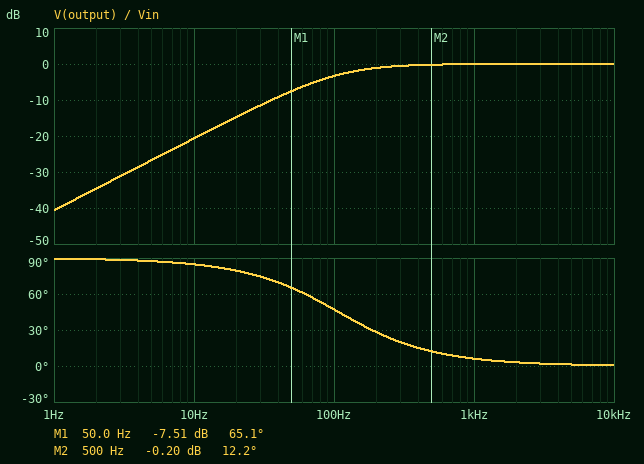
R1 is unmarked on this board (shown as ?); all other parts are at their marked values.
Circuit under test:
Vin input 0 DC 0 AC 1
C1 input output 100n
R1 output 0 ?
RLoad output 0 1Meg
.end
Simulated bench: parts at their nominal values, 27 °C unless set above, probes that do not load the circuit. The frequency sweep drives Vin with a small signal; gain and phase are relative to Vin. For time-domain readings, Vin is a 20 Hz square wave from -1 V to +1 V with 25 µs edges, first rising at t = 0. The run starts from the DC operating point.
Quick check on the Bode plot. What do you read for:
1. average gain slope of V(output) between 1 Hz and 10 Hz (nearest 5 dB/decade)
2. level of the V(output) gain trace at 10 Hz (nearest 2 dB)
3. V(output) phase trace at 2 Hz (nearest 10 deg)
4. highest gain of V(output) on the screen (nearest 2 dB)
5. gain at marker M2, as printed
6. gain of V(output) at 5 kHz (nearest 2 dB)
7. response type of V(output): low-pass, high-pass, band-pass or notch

20 dB/decade
-20 dB
90 deg
0 dB
-0.20 dB
0 dB
high-pass
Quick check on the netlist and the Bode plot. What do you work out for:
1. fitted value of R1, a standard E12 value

15 kΩ
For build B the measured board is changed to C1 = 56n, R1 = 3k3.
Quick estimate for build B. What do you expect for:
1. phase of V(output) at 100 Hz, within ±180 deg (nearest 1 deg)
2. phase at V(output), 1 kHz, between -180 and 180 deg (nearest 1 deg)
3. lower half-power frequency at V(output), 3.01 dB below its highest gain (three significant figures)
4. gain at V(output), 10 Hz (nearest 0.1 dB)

83 deg
41 deg
864 Hz
-38.7 dB
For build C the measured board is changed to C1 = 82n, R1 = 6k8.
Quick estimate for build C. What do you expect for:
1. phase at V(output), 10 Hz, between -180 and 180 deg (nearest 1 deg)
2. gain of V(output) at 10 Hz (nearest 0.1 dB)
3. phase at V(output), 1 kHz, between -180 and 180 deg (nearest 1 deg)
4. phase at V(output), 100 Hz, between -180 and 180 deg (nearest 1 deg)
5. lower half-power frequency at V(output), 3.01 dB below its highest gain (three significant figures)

88 deg
-29.2 dB
16 deg
71 deg
287 Hz
